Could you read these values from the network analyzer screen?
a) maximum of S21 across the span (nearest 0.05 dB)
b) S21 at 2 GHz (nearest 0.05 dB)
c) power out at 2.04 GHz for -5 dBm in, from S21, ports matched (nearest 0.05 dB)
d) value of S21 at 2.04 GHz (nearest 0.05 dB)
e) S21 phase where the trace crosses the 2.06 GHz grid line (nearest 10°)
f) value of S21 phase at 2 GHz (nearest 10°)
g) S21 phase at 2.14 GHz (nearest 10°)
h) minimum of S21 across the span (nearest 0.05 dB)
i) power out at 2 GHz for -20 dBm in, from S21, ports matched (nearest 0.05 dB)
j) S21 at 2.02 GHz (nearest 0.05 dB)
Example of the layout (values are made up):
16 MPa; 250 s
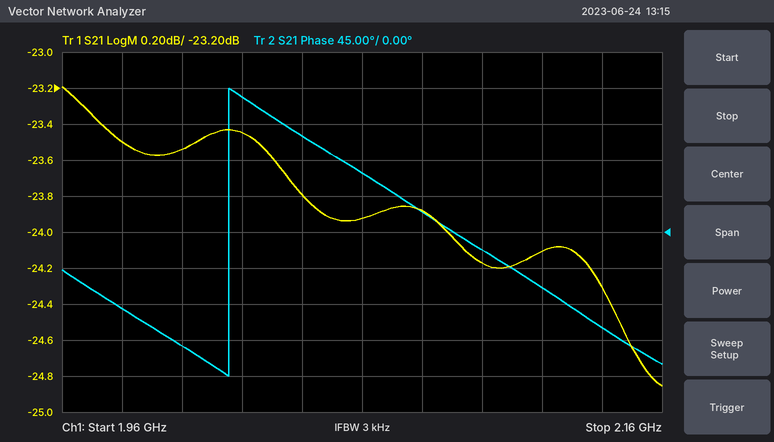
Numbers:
-23.20 dB; -23.55 dB; -28.80 dBm; -23.80 dB; 70°; -140°; -120°; -24.85 dB; -43.55 dBm; -23.45 dB
